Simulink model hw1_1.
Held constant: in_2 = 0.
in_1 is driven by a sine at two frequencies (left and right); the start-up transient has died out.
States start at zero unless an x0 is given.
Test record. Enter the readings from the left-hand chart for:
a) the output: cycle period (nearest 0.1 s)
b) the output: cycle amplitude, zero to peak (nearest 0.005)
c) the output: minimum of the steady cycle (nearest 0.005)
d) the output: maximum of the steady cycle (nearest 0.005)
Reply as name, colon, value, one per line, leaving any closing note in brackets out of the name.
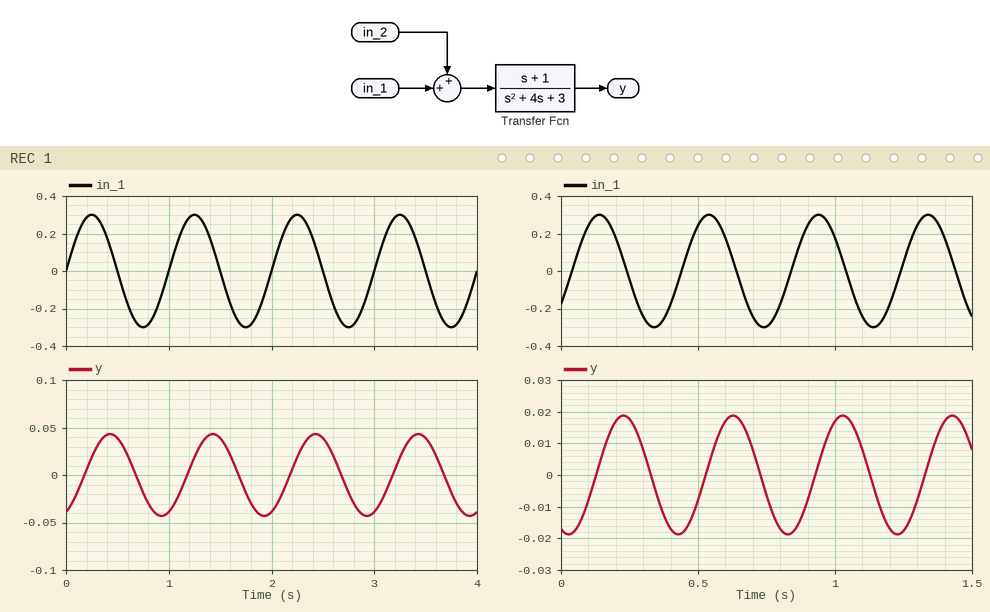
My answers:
the output: cycle period: 1.0 s
the output: cycle amplitude, zero to peak: 0.045
the output: minimum of the steady cycle: -0.045
the output: maximum of the steady cycle: 0.045
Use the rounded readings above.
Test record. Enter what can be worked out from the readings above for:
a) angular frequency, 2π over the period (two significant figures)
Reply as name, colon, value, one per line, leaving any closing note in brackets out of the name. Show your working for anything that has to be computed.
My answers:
angular frequency, 2π over the period: 2π / 1 = 6.3 rad/s
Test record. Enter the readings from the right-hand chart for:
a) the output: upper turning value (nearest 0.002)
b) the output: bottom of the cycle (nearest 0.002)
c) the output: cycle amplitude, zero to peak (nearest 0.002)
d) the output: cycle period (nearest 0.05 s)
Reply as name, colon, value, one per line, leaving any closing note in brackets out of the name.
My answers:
the output: upper turning value: 0.018
the output: bottom of the cycle: -0.018
the output: cycle amplitude, zero to peak: 0.018
the output: cycle period: 0.40 s
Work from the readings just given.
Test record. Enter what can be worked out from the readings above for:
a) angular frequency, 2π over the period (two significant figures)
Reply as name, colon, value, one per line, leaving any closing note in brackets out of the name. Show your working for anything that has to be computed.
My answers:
angular frequency, 2π over the period: 2π / 0.4 = 16 rad/s
